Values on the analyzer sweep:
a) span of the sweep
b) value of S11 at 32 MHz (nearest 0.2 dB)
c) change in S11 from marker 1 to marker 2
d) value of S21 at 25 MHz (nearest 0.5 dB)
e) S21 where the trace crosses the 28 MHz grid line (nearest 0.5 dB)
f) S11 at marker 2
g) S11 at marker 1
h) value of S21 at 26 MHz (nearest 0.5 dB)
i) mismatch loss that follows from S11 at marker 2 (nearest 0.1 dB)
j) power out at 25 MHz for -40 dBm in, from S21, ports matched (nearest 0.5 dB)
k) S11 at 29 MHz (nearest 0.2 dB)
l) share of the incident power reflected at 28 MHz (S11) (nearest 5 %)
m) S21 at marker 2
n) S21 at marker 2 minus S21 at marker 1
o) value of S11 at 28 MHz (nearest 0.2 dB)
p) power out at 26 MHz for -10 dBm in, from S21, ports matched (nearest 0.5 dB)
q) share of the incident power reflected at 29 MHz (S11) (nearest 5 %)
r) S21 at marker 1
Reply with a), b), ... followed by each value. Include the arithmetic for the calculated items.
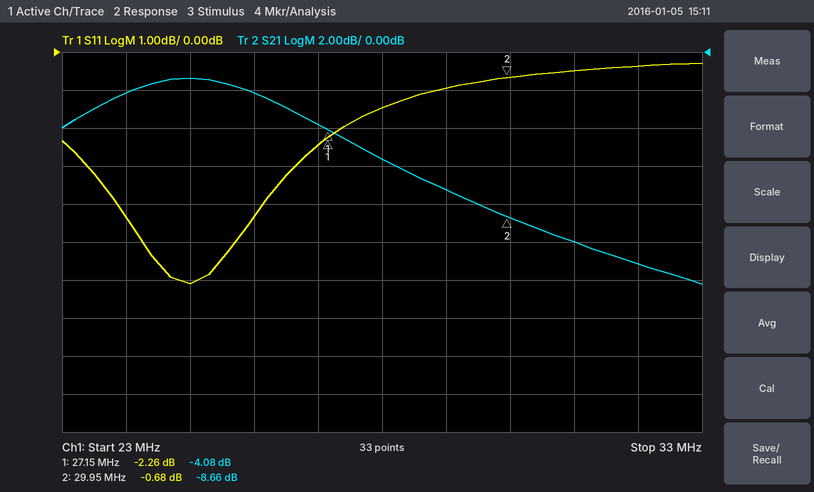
a) 10 MHz
b) -0.4 dB
c) -0.68 − (-2.26) = 1.58 dB
d) -1.5 dB
e) -5.5 dB
f) -0.68 dB
g) -2.26 dB
h) -2.0 dB
i) −10 log10(1 − 10^(-0.68/10)) ≈ 8.4 dB
j) -40 dBm + (-1.5 dB) = -41.5 dBm
k) -1.0 dB
l) 10^(-1.4/10) ≈ 72.4 %, so 70 % to the nearest 5 %
m) -8.66 dB
n) -8.66 − (-4.08) = -4.58 dB
o) -1.4 dB
p) -10 dBm + (-2.0 dB) = -12.0 dBm
q) 10^(-1/10) ≈ 79.4 %, so 80 % to the nearest 5 %
r) -4.08 dB
